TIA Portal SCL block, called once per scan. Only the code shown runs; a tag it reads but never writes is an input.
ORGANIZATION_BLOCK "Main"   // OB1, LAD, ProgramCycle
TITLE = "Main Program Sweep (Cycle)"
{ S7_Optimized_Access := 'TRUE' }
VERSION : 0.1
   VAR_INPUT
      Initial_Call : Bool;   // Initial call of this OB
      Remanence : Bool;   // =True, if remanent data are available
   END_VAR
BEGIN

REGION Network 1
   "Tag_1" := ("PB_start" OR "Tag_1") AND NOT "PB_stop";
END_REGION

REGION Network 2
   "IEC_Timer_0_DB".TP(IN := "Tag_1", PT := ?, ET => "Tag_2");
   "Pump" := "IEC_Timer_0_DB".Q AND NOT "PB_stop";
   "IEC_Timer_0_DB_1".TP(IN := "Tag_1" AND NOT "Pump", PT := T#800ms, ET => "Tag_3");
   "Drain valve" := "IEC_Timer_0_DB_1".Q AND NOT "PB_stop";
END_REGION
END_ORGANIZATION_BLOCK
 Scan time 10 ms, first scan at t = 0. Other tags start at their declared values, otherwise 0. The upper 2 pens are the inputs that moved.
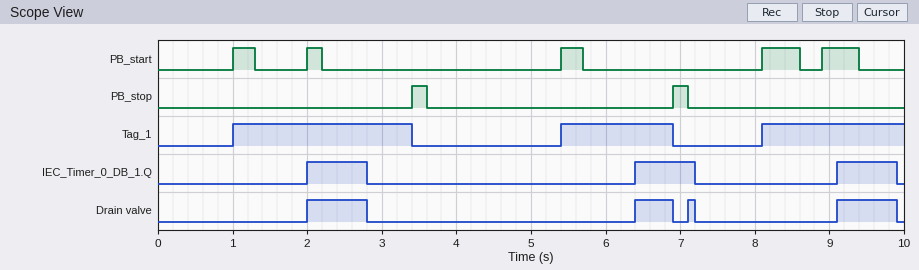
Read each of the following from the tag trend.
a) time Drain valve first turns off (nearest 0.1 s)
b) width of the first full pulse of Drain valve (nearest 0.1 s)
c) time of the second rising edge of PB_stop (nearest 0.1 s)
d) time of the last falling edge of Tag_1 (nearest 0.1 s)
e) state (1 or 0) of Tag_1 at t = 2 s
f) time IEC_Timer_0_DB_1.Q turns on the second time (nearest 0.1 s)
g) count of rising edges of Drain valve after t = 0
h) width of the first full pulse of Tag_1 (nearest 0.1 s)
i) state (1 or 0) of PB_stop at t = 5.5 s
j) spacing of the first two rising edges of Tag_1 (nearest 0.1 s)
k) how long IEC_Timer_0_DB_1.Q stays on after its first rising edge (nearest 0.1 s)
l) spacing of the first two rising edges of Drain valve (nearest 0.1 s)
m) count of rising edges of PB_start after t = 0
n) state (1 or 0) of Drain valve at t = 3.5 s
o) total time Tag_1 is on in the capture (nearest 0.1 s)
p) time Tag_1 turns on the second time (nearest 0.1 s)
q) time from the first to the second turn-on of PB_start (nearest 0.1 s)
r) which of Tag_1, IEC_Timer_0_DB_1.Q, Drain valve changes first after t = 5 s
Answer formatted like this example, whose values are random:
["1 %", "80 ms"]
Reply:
["2.8 s", "0.8 s", "6.9 s", "6.9 s", "1", "6.4 s", "4", "2.4 s", "0", "4.4 s", "0.8 s", "4.4 s", "5", "0", "5.8 s", "5.4 s", "1.0 s", "Tag_1"]
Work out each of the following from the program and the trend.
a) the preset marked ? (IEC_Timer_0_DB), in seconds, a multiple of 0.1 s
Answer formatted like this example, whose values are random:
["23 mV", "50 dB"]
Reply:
["1.0 s"]
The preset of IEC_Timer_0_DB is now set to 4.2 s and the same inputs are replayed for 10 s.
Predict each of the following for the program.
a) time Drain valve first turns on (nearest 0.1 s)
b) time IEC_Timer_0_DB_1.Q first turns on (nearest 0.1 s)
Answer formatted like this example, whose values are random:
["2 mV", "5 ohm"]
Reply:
["9.6 s", "9.6 s"]
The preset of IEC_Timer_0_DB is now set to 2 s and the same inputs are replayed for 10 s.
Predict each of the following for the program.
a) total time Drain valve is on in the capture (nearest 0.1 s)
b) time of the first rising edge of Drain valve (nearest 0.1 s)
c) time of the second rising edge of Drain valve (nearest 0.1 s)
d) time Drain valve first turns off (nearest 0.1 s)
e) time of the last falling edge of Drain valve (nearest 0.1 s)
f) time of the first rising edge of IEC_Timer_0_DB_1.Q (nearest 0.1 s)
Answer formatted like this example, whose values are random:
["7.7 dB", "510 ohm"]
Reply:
["0.6 s", "3.0 s", "3.6 s", "3.4 s", "3.8 s", "3.0 s"]
